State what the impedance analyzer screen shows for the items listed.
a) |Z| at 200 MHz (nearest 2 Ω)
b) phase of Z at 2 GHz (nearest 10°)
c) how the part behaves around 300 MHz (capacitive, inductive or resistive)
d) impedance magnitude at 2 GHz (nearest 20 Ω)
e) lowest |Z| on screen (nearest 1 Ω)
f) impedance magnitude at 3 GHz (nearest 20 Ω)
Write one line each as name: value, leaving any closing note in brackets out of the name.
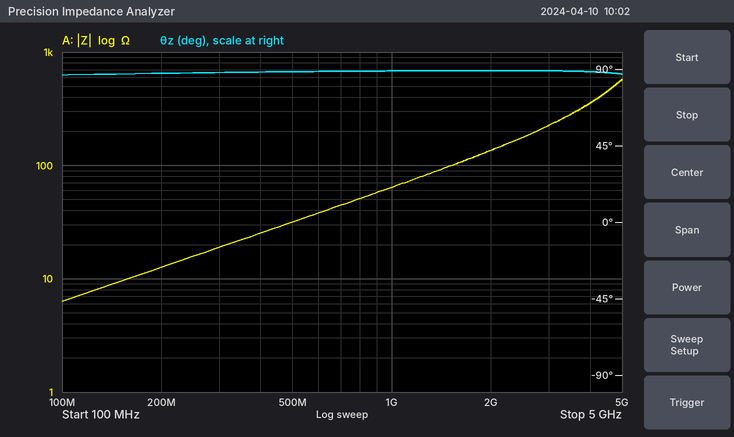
|Z| at 200 MHz: 12 Ω
phase of Z at 2 GHz: 90°
how the part behaves around 300 MHz: inductive
impedance magnitude at 2 GHz: 140 Ω
lowest |Z| on screen: 6 Ω
impedance magnitude at 3 GHz: 220 Ω
